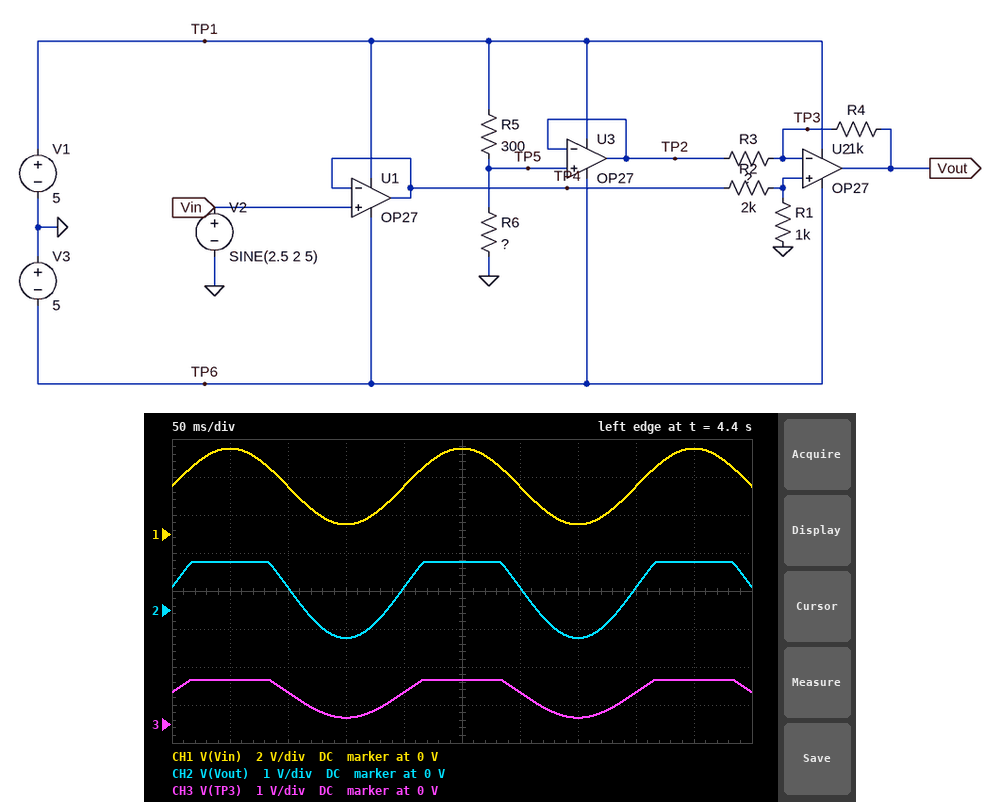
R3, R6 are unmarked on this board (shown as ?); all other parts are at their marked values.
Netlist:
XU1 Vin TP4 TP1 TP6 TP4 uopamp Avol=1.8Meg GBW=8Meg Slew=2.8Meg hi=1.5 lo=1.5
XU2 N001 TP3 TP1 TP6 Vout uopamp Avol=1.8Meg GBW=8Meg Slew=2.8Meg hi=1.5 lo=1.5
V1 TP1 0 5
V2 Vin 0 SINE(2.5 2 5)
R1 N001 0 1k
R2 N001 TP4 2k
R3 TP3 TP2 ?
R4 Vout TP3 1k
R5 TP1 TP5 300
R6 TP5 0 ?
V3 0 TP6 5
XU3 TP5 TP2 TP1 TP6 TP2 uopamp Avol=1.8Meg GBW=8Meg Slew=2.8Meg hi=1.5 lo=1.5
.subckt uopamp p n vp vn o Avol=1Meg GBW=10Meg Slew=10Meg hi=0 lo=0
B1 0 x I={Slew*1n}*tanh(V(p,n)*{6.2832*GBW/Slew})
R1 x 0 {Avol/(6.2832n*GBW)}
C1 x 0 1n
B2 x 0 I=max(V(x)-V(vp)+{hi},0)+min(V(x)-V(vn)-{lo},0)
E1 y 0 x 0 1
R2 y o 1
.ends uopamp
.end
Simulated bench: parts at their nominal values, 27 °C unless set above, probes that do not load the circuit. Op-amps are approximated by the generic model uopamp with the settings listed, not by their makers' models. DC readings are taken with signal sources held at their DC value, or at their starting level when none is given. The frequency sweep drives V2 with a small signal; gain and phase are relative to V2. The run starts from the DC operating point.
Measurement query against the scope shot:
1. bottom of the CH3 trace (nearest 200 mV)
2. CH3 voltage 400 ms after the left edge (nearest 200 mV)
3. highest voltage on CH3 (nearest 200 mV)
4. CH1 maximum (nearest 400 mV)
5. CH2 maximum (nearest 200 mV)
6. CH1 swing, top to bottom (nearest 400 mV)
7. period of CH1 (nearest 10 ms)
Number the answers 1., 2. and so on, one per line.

1. 200 mV
2. 800 mV
3. 1.2 V
4. 4.4 V
5. 1.2 V
6. 4.0 V
7. 200 ms
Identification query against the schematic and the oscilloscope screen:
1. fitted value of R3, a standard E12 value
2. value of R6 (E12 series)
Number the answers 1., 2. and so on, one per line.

1. 1 kΩ
2. 82 Ω
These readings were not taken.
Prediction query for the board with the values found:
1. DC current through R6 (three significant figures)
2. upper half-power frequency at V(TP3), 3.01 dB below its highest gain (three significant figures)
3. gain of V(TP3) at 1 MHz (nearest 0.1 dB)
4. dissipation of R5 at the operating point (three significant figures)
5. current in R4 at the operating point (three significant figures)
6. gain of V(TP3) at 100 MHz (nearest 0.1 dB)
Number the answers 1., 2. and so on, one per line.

1. 13.1 mA
2. 3.35 MHz
3. -9.9 dB
4. 51.4 mW
5. 240 µA
6. -59.5 dB
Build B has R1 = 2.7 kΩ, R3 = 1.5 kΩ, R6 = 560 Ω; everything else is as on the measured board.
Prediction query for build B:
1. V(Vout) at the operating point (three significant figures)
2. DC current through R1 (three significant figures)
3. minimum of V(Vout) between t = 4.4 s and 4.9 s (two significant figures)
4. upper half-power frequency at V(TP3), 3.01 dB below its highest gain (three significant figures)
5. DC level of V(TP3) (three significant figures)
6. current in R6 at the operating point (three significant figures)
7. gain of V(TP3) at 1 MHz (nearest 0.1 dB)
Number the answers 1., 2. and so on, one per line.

1. 223 mV
2. 532 µA
3. -1.7 V
4. 3.81 MHz
5. 1.44 V
6. 5.81 mA
7. -5.1 dB
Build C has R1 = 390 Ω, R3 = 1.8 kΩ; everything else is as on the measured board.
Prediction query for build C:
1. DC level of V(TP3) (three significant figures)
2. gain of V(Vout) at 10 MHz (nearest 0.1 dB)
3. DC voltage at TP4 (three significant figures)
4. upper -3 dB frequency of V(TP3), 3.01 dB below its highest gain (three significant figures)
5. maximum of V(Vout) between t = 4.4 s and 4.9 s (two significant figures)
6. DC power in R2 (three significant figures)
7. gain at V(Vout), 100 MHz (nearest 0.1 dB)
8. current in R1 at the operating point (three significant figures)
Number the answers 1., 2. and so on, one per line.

1. 408 mV
2. -22.8 dB
3. 2.50 V
4. 3.99 MHz
5. 290 mV
6. 2.19 mW
7. -59.7 dB
8. 1.05 mA
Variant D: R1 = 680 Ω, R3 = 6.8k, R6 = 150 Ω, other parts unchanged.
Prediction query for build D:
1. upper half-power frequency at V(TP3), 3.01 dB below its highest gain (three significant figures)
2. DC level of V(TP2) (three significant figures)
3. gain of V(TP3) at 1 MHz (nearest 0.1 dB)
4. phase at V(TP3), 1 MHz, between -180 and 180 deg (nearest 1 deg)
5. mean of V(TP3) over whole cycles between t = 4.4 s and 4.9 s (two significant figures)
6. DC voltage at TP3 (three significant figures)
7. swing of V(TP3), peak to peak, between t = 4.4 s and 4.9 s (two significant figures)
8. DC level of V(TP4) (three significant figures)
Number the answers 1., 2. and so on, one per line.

1. 4.79 MHz
2. 1.67 V
3. -12.1 dB
4. -15 deg
5. 580 mV
6. 634 mV
7. 760 mV
8. 2.50 V
